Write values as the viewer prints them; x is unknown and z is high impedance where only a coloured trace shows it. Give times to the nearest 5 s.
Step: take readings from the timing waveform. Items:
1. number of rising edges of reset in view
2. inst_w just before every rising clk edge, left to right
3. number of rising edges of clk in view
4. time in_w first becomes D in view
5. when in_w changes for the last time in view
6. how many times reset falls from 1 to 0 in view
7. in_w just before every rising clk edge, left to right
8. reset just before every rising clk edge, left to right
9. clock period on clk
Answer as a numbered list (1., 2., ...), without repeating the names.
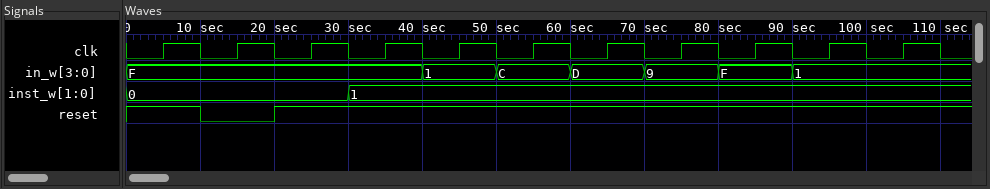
1. 1
2. 0, 0, 0, 1, 1, 1, 1, 1, 1, 1, 1
3. 11
4. 60 s
5. 90 s
6. 1
7. F, F, F, F, 1, C, D, 9, F, 1, 1
8. 1 0 1 1 1 1 1 1 1 1 1
9. 10 s
